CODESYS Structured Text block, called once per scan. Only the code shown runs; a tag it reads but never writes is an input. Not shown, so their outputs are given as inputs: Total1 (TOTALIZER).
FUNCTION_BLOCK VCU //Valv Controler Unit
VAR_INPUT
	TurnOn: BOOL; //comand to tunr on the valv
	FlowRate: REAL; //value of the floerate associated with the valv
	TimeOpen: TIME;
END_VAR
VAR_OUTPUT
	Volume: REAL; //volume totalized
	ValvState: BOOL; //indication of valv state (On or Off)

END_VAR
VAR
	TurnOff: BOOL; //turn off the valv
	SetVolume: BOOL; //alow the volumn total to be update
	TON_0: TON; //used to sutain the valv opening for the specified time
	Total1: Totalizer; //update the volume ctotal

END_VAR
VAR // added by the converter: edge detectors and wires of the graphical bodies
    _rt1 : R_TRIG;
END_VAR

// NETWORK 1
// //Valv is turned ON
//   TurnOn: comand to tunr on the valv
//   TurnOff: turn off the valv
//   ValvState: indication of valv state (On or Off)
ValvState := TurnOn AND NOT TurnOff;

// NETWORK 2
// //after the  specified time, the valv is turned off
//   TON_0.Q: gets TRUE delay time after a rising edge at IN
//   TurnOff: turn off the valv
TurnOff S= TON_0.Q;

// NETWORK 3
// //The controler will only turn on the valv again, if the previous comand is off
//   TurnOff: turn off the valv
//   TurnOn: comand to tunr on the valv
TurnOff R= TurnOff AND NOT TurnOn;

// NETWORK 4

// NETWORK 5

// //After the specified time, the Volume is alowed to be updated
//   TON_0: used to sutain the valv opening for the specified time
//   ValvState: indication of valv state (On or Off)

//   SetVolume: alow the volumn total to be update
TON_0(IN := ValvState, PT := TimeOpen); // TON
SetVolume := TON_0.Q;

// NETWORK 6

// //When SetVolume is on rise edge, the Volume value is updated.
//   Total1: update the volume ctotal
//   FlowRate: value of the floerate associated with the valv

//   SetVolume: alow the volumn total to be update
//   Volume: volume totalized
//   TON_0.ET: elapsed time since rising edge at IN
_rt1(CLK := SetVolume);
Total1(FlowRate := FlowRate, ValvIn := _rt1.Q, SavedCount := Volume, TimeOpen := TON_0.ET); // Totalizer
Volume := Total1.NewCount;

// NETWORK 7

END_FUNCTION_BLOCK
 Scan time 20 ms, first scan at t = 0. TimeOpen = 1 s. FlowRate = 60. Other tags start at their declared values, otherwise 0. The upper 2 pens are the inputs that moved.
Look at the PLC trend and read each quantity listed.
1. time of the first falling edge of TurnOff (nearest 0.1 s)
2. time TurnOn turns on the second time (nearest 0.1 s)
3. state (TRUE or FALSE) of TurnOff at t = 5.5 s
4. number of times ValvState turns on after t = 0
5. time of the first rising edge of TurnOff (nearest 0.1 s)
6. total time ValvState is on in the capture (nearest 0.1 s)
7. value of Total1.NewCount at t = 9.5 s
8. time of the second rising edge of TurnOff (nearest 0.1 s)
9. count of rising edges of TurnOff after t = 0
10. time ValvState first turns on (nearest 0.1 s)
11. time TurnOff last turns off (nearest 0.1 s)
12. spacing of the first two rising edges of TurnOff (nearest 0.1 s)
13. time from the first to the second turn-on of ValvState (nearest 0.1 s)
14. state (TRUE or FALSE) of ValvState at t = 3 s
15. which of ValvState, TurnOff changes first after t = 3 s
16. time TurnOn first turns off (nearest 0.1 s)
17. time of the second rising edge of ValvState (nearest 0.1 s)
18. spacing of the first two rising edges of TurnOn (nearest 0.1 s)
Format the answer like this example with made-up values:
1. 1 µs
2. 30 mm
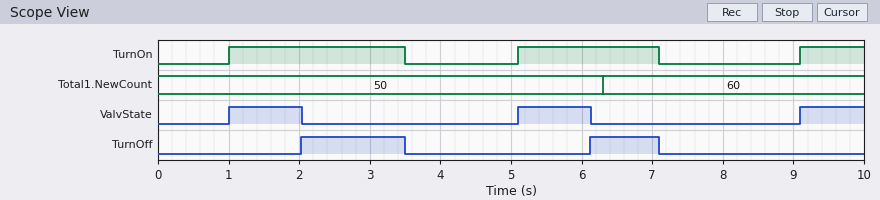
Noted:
1. 3.5 s
2. 5.1 s
3. FALSE
4. 3
5. 2.0 s
6. 3.0 s
7. 60
8. 6.1 s
9. 2
10. 1.0 s
11. 7.1 s
12. 4.1 s
13. 4.1 s
14. FALSE
15. TurnOff
16. 3.5 s
17. 5.1 s
18. 4.1 s
